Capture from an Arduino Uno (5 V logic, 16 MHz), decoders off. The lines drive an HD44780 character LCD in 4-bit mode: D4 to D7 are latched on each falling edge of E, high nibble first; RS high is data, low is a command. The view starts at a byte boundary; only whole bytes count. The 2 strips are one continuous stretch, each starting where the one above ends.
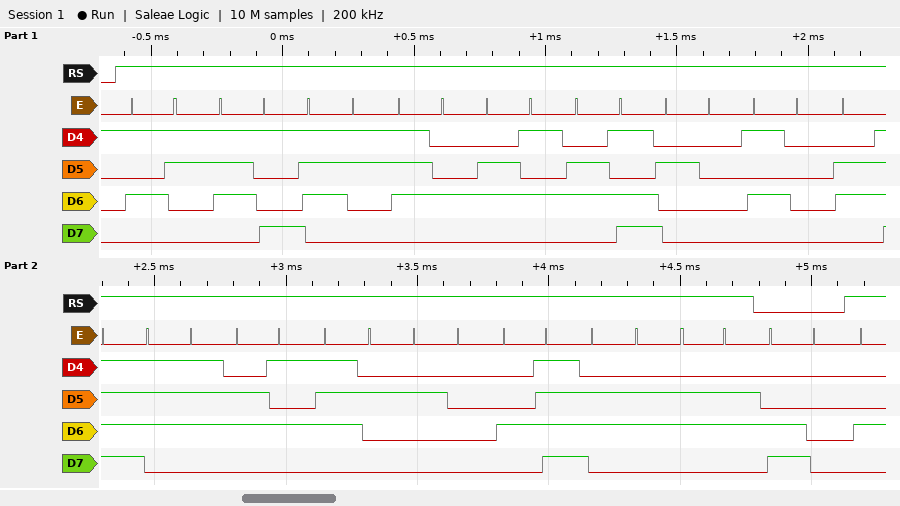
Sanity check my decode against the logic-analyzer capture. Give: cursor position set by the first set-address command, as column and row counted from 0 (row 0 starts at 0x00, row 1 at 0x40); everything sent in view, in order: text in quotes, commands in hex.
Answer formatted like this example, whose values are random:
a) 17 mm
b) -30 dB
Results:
a) column 0, row 1
b) "System Power Off" 0xC0
